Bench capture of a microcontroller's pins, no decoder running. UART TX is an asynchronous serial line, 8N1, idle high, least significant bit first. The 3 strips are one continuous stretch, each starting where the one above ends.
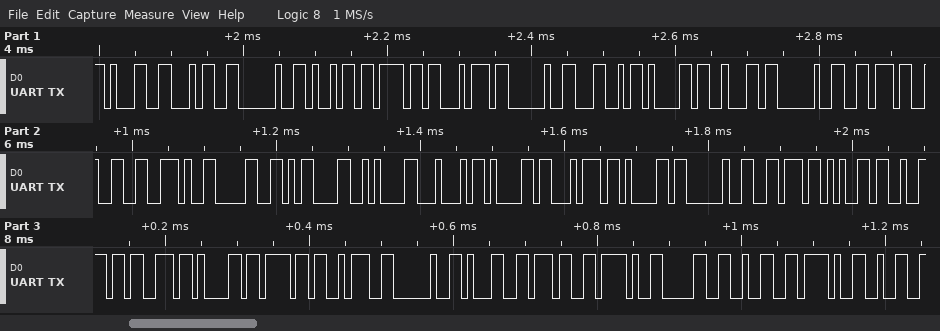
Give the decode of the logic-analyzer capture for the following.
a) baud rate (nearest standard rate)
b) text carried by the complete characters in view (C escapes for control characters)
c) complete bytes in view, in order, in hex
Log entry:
115200 baud
"14 iot Lab v2.0\r\nData versao: 17/02/2"
31 34 20 69 6F 74 20 4C 61 62 20 76 32 2E 30 0D 0A 44 61 74 61 20 76 65 72 73 61 6F 3A 20 31 37 2F 30 32 2F 32
